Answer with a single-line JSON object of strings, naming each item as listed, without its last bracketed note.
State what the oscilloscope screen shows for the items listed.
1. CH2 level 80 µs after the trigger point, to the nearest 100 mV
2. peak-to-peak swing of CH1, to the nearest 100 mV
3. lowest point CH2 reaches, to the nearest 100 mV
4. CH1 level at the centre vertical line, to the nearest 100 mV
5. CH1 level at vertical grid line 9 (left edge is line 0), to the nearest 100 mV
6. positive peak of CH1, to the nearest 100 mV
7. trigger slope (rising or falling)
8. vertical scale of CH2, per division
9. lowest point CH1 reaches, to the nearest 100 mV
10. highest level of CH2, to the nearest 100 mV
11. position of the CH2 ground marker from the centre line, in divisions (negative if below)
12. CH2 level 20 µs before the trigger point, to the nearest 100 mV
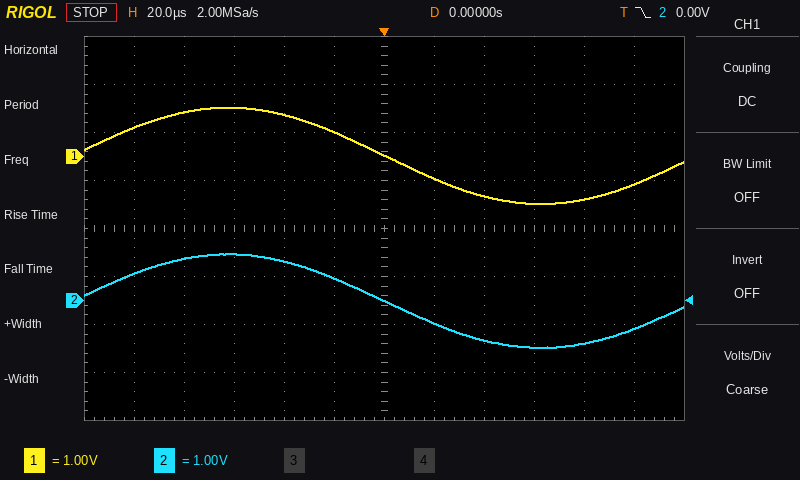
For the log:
{"CH2 level 80 µs after the trigger point, to the nearest 100 mV": "-900 mV", "peak-to-peak swing of CH1, to the nearest 100 mV": "2.0 V", "lowest point CH2 reaches, to the nearest 100 mV": "-1.0 V", "CH1 level at the centre vertical line, to the nearest 100 mV": "0.0 V", "CH1 level at vertical grid line 9 (left edge is line 0), to the nearest 100 mV": "-1.0 V", "positive peak of CH1, to the nearest 100 mV": "1.0 V", "trigger slope": "falling", "vertical scale of CH2, per division": "1 V", "lowest point CH1 reaches, to the nearest 100 mV": "-1.0 V", "highest level of CH2, to the nearest 100 mV": "1.0 V", "position of the CH2 ground marker from the centre line, in divisions": "-1.5 div", "CH2 level 20 µs before the trigger point, to the nearest 100 mV": "500 mV"}
